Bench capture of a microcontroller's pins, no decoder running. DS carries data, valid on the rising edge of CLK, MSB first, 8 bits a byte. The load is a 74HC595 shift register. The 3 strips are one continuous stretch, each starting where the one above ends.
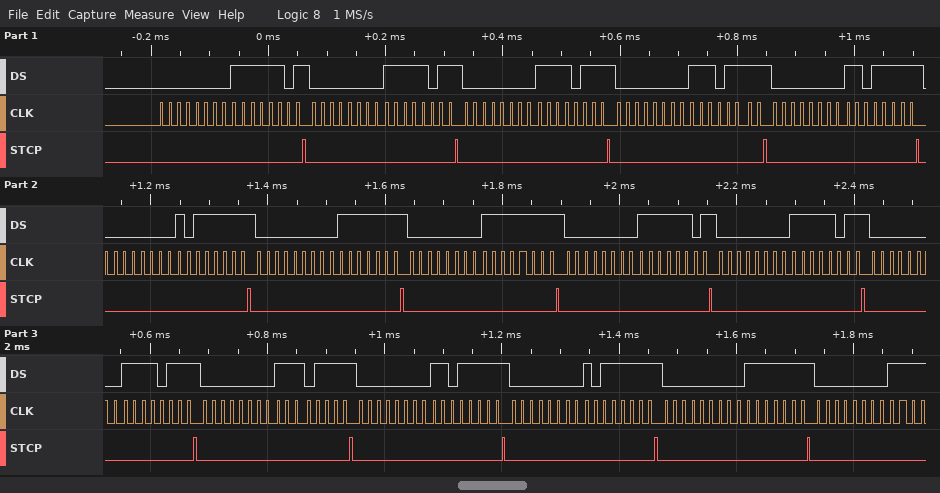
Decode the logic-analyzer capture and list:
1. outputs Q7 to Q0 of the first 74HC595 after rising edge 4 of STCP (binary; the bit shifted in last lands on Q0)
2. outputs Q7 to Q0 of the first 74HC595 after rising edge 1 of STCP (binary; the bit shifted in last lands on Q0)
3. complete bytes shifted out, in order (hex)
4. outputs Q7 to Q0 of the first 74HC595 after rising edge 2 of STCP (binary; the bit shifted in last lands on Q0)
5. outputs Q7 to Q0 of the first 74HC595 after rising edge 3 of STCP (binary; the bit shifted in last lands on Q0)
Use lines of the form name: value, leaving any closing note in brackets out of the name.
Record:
outputs Q7 to Q0 of the first 74HC595 after rising edge 4 of STCP: 11101111
outputs Q7 to Q0 of the first 74HC595 after rising edge 1 of STCP: 11111101
complete bytes shifted out, in order: 00 FD 00 FB 00 F7 00 EF 00 DF 00 BF 00 7F 00 FF 00 FD 00 FB 00 F7 00 EF 00 DF 00 BF 00 7F 00
outputs Q7 to Q0 of the first 74HC595 after rising edge 2 of STCP: 11111011
outputs Q7 to Q0 of the first 74HC595 after rising edge 3 of STCP: 11110111
